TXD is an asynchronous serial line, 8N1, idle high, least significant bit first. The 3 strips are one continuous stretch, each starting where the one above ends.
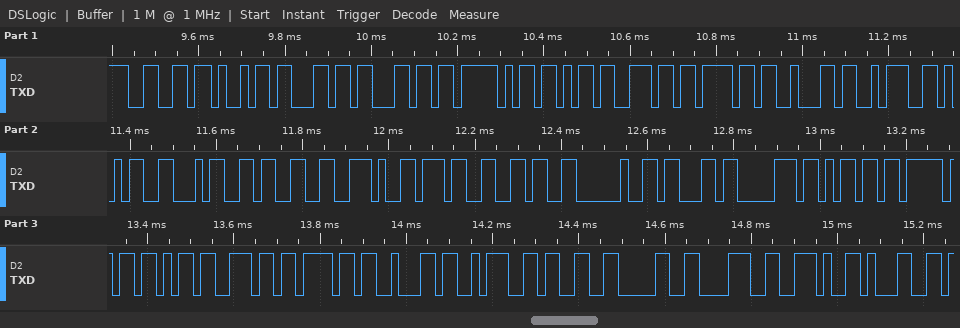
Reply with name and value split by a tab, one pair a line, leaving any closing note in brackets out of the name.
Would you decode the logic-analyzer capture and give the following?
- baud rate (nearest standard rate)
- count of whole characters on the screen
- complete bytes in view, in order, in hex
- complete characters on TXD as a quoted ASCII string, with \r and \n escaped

baud rate	57600 baud
count of whole characters on the screen	31
complete bytes in view, in order, in hex	66 69 6C 6C 5F 6B 6E 6F 62 3A 35 34 33 2E 37 36 20 63 70 6D 5F 6B 6E 6F 62 3A 33 30 38 2E 31
complete characters on TXD as a quoted ASCII string, with \r and \n escaped	"fill_knob:543.76 cpm_knob:308.1"
